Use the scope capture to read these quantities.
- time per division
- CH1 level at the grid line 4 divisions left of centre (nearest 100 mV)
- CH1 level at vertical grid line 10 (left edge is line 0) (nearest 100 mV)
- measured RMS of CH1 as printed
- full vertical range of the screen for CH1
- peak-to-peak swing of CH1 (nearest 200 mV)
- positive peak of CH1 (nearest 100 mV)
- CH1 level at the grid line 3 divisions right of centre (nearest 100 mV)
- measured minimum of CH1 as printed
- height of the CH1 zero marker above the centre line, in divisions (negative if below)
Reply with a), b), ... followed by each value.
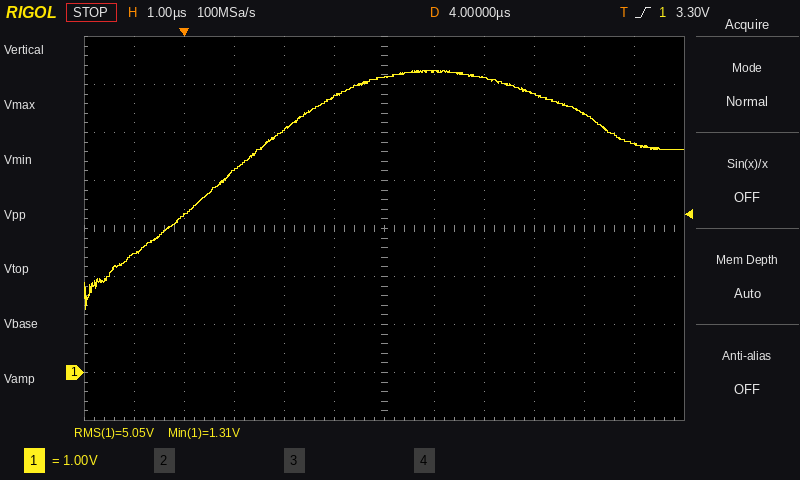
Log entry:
a) 1 µs
b) 3.3 V
c) 5.4 V
d) 5.05 V
e) 8 V
f) 5.0 V
g) 6.3 V
h) 5.8 V
i) 1.31 V
j) -3.0 div
